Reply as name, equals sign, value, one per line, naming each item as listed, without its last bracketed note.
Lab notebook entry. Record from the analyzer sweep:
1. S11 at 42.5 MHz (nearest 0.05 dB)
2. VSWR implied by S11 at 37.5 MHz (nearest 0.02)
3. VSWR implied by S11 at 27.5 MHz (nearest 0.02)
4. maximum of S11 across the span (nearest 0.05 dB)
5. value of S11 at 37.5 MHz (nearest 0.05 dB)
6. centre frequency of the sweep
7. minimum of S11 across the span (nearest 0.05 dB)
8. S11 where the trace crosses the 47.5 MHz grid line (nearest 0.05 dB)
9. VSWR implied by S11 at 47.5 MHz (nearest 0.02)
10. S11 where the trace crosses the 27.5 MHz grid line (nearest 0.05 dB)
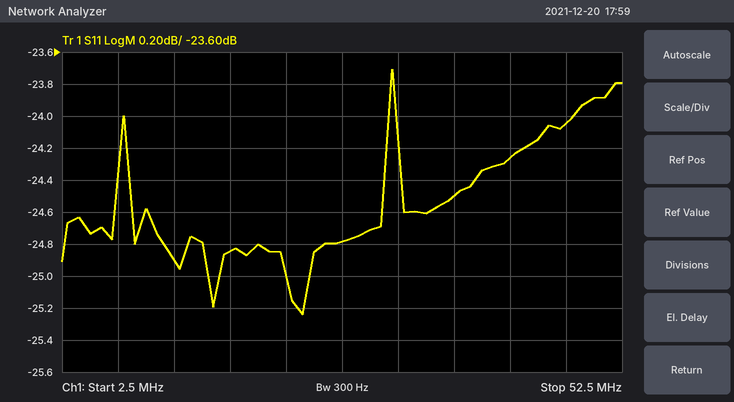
S11 at 42.5 MHz = -24.25 dB
VSWR implied by S11 at 37.5 MHz = 1.12
VSWR implied by S11 at 27.5 MHz = 1.12
maximum of S11 across the span = -23.70 dB
value of S11 at 37.5 MHz = -24.50 dB
centre frequency of the sweep = 27.5 MHz
minimum of S11 across the span = -25.25 dB
S11 where the trace crosses the 47.5 MHz grid line = -24.05 dB
VSWR implied by S11 at 47.5 MHz = 1.14
S11 where the trace crosses the 27.5 MHz grid line = -24.80 dB
